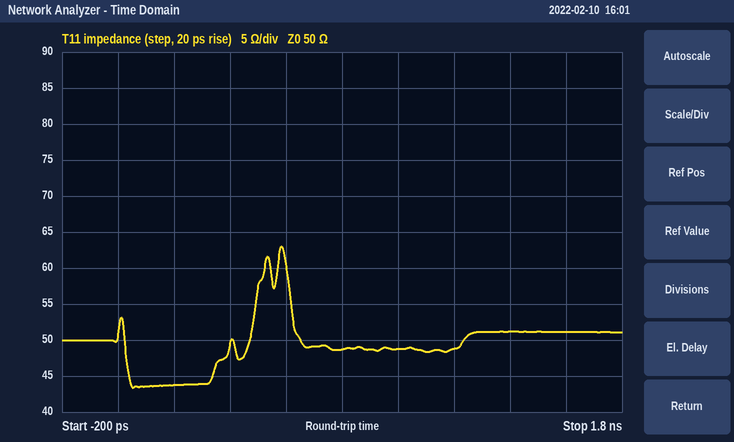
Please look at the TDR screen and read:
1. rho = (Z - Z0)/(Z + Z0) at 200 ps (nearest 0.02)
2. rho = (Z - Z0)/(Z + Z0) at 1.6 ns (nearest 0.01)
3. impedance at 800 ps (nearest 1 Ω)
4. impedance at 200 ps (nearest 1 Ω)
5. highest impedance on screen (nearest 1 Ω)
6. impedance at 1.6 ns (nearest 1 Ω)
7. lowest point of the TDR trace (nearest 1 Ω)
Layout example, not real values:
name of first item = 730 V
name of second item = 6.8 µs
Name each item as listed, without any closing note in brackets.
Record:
rho = (Z - Z0)/(Z + Z0) at 200 ps = -0.06
rho = (Z - Z0)/(Z + Z0) at 1.6 ns = +0.01
impedance at 800 ps = 49 Ω
impedance at 200 ps = 44 Ω
highest impedance on screen = 63 Ω
impedance at 1.6 ns = 51 Ω
lowest point of the TDR trace = 43 Ω
